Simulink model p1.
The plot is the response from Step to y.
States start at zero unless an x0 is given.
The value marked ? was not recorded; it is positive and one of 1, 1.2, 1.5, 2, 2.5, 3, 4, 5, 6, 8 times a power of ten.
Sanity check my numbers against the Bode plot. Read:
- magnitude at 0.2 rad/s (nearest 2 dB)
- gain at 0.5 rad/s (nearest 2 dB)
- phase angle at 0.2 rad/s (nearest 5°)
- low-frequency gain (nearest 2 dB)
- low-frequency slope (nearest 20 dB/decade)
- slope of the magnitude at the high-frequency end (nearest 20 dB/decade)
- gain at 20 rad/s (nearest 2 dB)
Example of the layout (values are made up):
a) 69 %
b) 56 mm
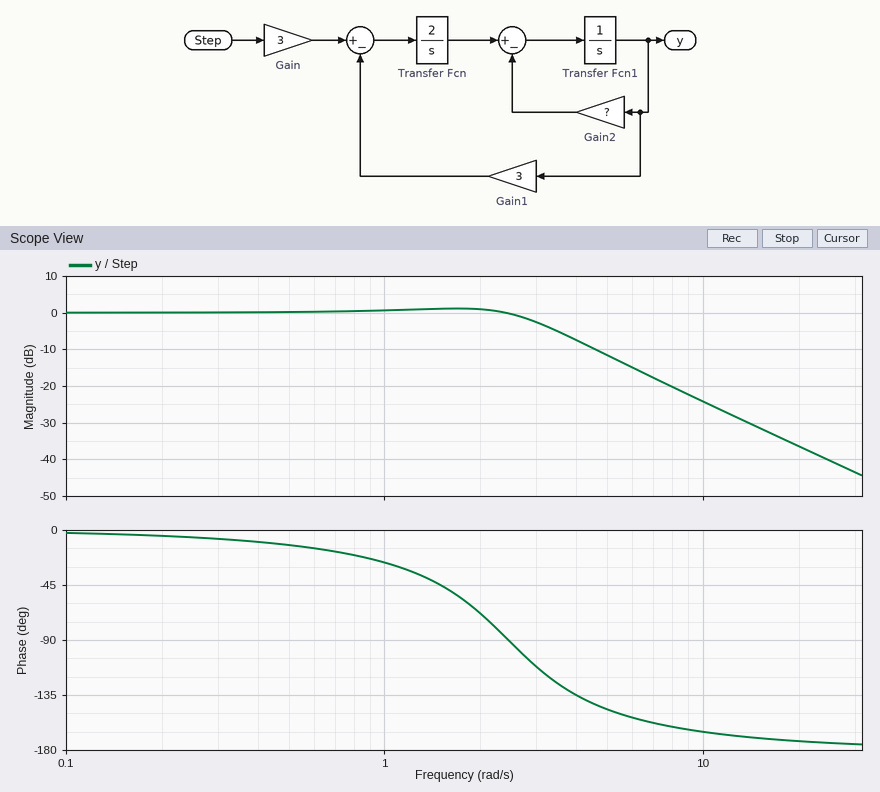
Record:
a) 0 dB
b) 0 dB
c) -5°
d) 0 dB
e) 0 dB/decade
f) -40 dB/decade
g) -36 dB
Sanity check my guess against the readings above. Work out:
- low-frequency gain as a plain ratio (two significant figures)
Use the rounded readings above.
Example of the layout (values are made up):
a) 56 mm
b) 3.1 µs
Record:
a) 1.0
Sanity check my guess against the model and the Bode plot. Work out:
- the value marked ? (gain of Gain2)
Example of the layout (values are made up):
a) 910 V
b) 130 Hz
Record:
a) 2.5
